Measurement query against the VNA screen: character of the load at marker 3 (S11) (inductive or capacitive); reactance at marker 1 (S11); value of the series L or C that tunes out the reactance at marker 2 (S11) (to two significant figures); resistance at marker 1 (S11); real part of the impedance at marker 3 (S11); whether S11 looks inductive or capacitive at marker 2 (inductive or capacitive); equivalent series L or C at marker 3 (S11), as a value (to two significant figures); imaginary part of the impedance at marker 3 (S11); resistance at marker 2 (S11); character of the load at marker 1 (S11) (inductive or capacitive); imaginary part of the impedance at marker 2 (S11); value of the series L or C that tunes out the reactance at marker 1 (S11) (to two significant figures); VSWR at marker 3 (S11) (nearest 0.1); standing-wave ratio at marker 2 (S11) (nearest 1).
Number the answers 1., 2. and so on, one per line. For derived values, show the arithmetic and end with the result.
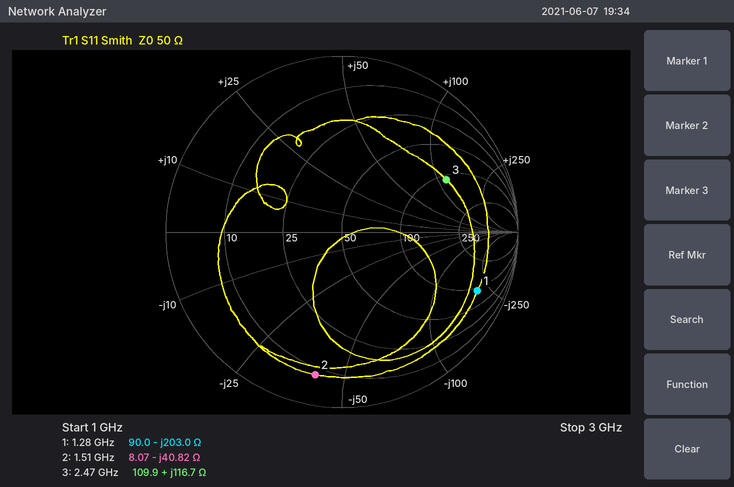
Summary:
1. inductive
2. -203.0 Ω
3. L = 40.82 Ω/(2π × 1.51 GHz) ≈ 4.3 nH
4. 90.0 Ω
5. 109.9 Ω
6. capacitive
7. L = 116.7 Ω/(2π × 2.47 GHz) ≈ 7.5 nH
8. +116.7 Ω
9. 8.07 Ω
10. capacitive
11. -40.82 Ω
12. L = 203 Ω/(2π × 1.28 GHz) ≈ 25 nH
13. 4.9
14. 10
